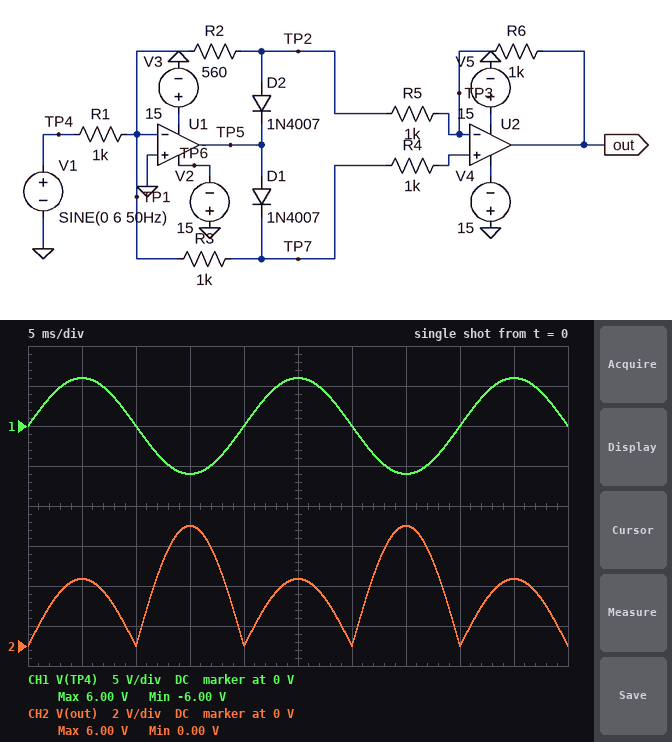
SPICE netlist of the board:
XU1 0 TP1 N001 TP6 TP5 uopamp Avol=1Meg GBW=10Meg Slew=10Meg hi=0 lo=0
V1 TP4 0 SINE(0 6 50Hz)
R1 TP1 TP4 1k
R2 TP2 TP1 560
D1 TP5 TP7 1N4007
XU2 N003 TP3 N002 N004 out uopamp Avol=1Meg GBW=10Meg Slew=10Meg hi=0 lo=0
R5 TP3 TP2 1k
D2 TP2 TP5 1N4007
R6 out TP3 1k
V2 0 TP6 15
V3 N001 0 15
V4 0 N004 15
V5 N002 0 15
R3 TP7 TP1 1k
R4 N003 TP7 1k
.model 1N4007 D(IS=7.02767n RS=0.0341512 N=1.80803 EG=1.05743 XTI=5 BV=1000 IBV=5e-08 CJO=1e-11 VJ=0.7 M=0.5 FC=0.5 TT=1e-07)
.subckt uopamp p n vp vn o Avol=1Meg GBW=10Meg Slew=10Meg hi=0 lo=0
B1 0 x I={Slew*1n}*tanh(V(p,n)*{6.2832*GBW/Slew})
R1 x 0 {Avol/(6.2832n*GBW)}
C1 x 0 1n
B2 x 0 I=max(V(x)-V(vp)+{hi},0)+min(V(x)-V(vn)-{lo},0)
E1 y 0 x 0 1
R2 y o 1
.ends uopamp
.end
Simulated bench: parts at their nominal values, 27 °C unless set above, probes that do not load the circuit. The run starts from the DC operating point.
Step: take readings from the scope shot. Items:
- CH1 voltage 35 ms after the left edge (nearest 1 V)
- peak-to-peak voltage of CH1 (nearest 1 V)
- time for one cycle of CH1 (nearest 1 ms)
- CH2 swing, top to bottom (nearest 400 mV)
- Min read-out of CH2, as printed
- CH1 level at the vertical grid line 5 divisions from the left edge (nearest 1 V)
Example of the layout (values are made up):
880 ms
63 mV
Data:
-6 V
12 V
20 ms
6.0 V
0.00 V
6 V
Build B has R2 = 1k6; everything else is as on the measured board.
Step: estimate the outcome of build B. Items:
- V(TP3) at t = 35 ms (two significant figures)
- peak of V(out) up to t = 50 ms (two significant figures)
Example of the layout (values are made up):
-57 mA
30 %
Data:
4.3 V
9.6 V
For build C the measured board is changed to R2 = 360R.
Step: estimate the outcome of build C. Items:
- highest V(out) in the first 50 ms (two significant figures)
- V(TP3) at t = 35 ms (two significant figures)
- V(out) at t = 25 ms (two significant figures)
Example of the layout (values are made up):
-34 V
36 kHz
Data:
6.0 V
3.5 V
2.2 V
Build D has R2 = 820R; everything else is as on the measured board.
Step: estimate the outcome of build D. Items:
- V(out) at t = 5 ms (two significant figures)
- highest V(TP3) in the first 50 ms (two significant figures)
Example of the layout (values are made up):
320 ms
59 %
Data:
4.9 V
3.9 V
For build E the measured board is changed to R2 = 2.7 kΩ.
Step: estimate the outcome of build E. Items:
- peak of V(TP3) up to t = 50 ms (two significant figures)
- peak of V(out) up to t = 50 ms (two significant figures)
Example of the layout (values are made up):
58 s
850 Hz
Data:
4.7 V
15 V
